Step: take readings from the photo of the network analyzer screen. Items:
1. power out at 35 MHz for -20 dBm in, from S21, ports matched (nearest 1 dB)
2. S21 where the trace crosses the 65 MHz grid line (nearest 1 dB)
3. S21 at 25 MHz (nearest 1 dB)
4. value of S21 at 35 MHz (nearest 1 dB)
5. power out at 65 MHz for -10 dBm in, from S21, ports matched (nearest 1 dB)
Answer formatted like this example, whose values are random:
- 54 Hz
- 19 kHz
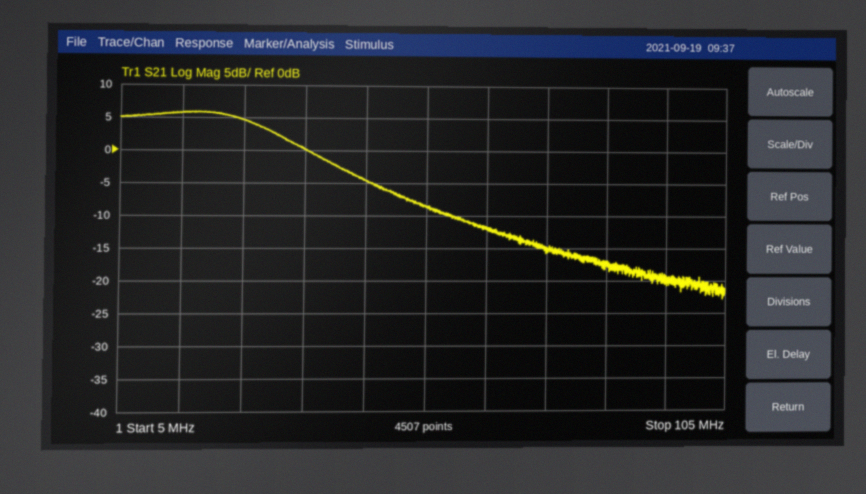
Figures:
- -20 dBm
- -12 dB
- 5 dB
- 0 dB
- -22 dBm
